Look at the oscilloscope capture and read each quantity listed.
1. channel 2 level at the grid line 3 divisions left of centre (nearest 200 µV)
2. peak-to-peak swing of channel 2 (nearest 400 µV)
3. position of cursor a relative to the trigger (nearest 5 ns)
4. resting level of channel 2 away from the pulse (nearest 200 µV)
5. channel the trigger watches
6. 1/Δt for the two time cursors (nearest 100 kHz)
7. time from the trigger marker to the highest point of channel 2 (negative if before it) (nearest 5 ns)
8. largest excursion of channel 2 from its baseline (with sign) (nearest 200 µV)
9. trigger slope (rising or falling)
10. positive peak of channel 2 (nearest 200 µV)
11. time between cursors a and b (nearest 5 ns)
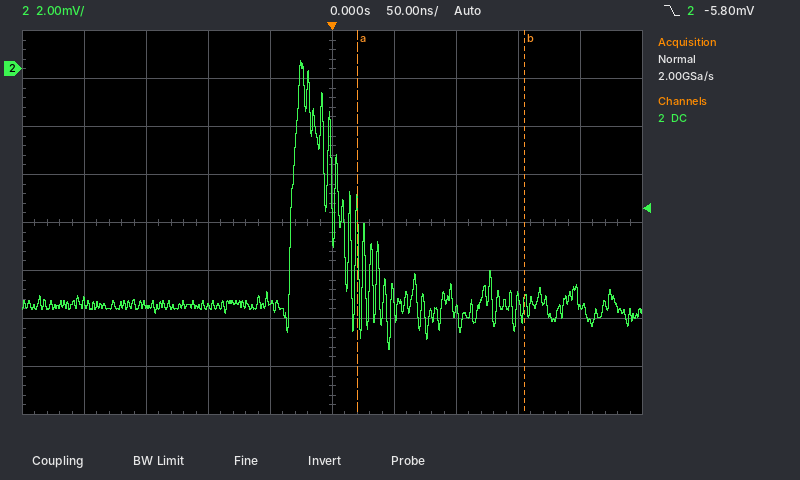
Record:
-9.8 mV
12.0 mV
+20 ns
-9.8 mV
channel 2
7.4 MHz
-25 ns
+10.2 mV
falling
400 µV
135 ns
